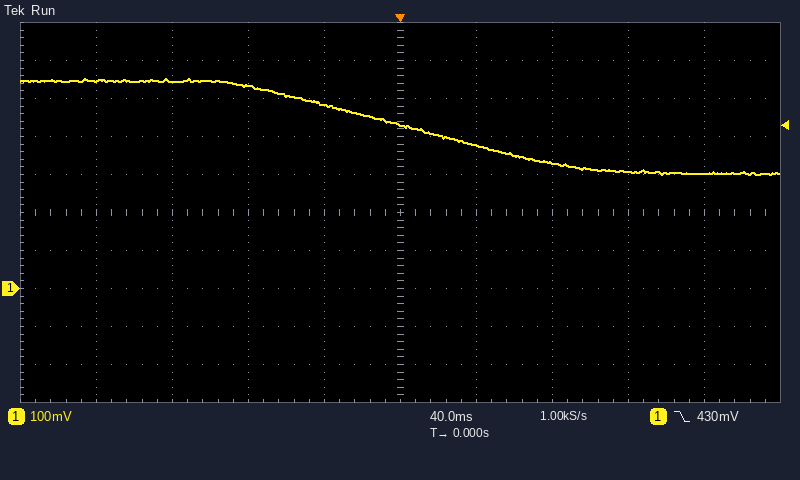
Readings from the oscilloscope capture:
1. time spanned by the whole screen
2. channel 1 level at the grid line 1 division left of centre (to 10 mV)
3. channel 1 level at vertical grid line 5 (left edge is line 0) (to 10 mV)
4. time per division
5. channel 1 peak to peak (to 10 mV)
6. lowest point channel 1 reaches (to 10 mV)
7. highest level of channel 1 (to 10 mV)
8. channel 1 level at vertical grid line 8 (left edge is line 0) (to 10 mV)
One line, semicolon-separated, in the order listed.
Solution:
400 ms; 480 mV; 430 mV; 40 ms; 250 mV; 300 mV; 550 mV; 310 mV
